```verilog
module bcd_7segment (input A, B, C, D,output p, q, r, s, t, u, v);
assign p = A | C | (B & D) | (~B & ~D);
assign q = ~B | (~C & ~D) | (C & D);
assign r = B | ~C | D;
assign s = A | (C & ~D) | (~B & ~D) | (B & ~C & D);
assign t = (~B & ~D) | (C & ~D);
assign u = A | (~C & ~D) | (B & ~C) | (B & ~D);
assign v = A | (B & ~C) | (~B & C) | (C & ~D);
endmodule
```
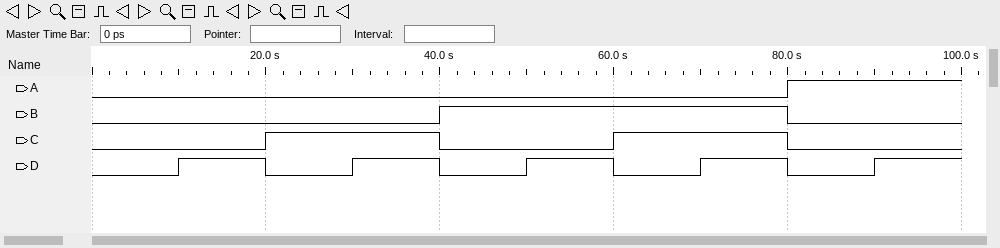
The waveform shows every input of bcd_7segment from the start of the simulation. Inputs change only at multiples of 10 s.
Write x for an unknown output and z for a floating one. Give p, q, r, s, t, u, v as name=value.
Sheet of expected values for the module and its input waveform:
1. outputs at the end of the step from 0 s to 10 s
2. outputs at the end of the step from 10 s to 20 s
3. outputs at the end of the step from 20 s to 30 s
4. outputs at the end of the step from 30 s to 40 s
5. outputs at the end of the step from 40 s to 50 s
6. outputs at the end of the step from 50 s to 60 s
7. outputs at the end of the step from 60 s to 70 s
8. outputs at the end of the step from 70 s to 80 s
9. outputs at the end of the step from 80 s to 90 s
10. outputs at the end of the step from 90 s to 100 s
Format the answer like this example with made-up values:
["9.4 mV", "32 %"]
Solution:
["p=1, q=1, r=1, s=1, t=1, u=1, v=0", "p=0, q=1, r=1, s=0, t=0, u=0, v=0", "p=1, q=1, r=0, s=1, t=1, u=0, v=1", "p=1, q=1, r=1, s=0, t=0, u=0, v=1", "p=0, q=1, r=1, s=0, t=0, u=1, v=1", "p=1, q=0, r=1, s=1, t=0, u=1, v=1", "p=1, q=0, r=1, s=1, t=1, u=1, v=1", "p=1, q=1, r=1, s=0, t=0, u=0, v=0", "p=1, q=1, r=1, s=1, t=1, u=1, v=1", "p=1, q=1, r=1, s=1, t=0, u=1, v=1"]
